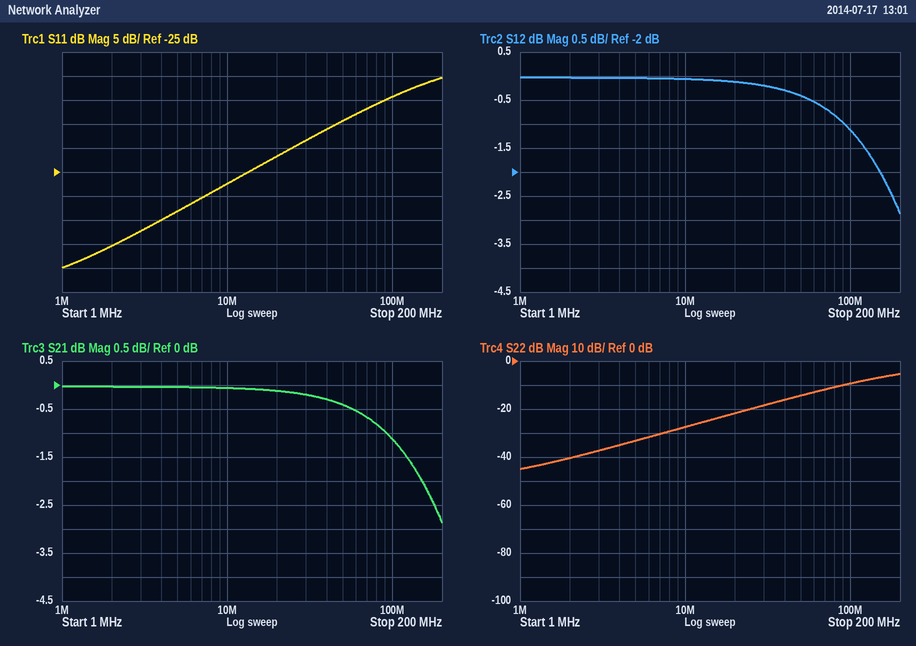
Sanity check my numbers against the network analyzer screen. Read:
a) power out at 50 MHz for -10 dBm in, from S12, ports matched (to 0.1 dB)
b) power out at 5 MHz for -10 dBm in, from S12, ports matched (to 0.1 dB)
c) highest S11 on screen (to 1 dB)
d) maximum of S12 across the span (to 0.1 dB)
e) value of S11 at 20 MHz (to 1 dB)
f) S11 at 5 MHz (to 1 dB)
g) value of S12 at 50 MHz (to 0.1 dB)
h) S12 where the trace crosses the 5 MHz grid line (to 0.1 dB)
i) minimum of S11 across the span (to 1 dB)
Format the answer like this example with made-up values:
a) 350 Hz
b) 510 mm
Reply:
a) -10.4 dBm
b) -10.0 dBm
c) -5 dB
d) 0.0 dB
e) -22 dB
f) -33 dB
g) -0.4 dB
h) 0.0 dB
i) -45 dB
